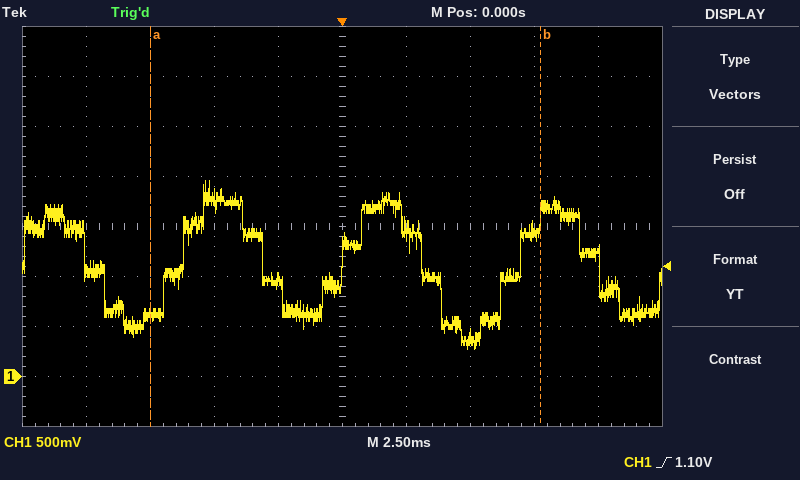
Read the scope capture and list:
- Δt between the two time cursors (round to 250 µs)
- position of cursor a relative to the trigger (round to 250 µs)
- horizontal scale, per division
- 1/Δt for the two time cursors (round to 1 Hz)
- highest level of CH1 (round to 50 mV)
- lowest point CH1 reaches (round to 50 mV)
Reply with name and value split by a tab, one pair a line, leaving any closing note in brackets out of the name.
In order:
Δt between the two time cursors	15.25 ms
position of cursor a relative to the trigger	-7.50 ms
horizontal scale, per division	2.5 ms
1/Δt for the two time cursors	66 Hz
highest level of CH1	1.95 V
lowest point CH1 reaches	300 mV
